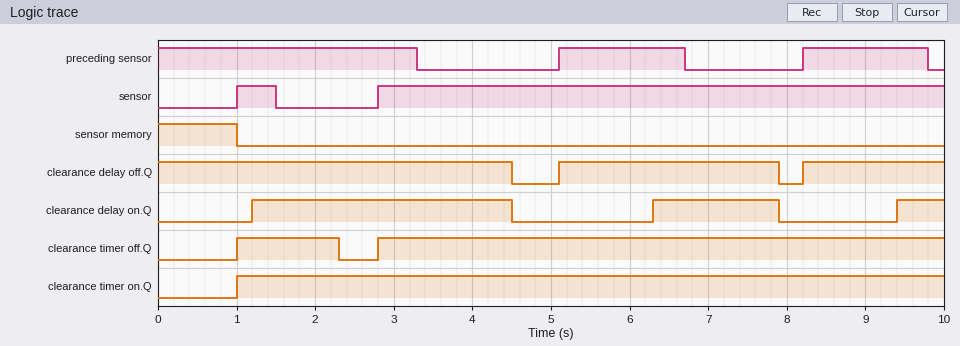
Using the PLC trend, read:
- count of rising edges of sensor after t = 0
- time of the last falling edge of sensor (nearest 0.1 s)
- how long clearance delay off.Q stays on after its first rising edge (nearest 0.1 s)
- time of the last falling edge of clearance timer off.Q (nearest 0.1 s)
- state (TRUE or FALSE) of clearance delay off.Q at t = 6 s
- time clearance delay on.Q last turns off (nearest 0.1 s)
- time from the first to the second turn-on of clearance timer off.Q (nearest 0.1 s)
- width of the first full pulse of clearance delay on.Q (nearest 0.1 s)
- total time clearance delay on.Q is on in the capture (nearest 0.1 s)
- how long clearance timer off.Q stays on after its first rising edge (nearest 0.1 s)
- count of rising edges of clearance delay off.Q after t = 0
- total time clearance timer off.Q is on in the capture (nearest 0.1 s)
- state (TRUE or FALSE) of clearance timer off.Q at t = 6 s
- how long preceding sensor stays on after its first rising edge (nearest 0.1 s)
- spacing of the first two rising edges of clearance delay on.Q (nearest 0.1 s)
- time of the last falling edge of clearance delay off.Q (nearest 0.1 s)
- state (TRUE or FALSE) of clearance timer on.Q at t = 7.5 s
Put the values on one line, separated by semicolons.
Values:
2; 1.5 s; 2.8 s; 2.3 s; TRUE; 7.9 s; 1.8 s; 3.3 s; 5.5 s; 1.3 s; 2; 8.5 s; TRUE; 1.6 s; 5.1 s; 7.9 s; TRUE
